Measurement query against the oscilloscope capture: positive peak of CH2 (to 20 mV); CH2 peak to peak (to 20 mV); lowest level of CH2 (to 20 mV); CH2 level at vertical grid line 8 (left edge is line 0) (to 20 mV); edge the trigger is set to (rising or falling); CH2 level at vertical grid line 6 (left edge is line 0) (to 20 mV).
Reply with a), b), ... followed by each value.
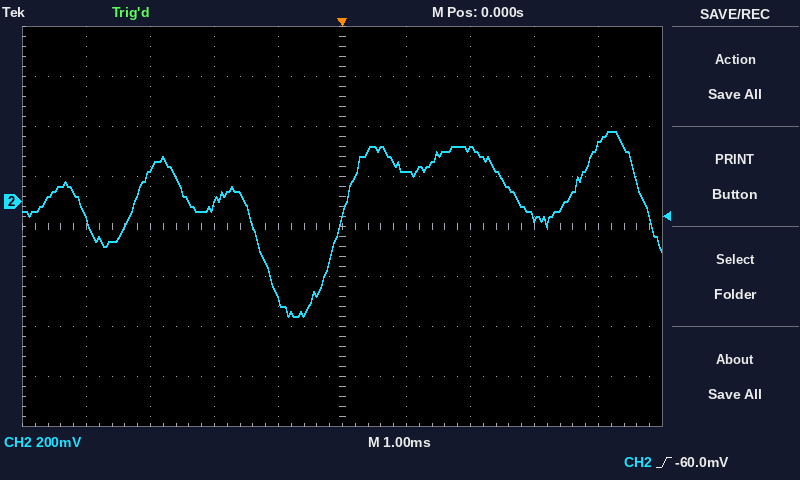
a) 280 mV
b) 740 mV
c) -460 mV
d) -60 mV
e) rising
f) 120 mV
